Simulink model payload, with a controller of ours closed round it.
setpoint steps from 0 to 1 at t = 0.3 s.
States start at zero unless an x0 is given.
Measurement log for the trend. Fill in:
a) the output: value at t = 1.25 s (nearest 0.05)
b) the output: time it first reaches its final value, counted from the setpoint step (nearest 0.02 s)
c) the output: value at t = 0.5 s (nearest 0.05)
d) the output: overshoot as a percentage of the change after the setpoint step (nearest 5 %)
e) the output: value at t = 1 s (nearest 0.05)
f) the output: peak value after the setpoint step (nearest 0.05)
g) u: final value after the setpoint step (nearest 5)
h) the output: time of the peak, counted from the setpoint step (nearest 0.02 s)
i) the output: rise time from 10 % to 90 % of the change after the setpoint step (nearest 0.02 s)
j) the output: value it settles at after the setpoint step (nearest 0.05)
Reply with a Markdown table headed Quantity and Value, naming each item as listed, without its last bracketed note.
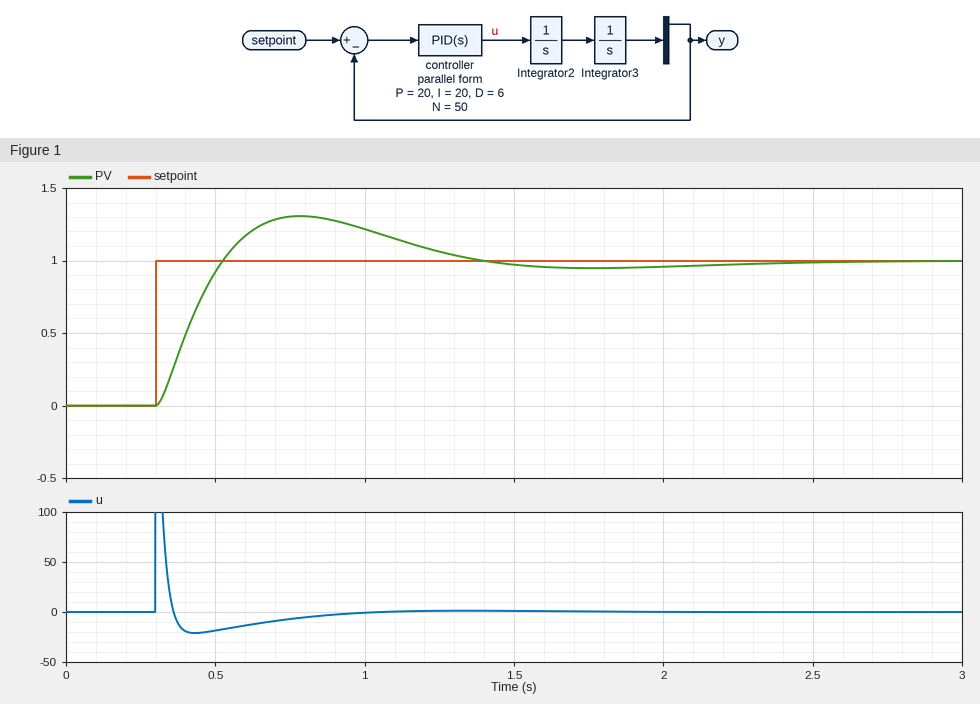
| Quantity | Value |
|---|---|
| the output: value at t = 1.25 s | 1.05 |
| the output: time it first reaches its final value, counted from the setpoint step | 0.22 s |
| the output: value at t = 0.5 s | 0.90 |
| the output: overshoot as a percentage of the change after the setpoint step | 30 % |
| the output: value at t = 1 s | 1.20 |
| the output: peak value after the setpoint step | 1.30 |
| u: final value after the setpoint step | 0 |
| the output: time of the peak, counted from the setpoint step | 0.48 s |
| the output: rise time from 10 % to 90 % of the change after the setpoint step | 0.16 s |
| the output: value it settles at after the setpoint step | 1.00 |
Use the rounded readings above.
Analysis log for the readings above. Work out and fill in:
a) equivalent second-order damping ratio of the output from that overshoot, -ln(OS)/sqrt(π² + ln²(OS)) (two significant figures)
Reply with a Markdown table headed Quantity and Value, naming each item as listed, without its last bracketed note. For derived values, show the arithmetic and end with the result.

| Quantity | Value |
|---|---|
| equivalent second-order damping ratio of the output from that overshoot, -ln(OS)/sqrt(π² + ln²(OS)) | ln(0.3) = -1.204; 1.204 / sqrt(9.870 + 1.450) = 0.36 |
